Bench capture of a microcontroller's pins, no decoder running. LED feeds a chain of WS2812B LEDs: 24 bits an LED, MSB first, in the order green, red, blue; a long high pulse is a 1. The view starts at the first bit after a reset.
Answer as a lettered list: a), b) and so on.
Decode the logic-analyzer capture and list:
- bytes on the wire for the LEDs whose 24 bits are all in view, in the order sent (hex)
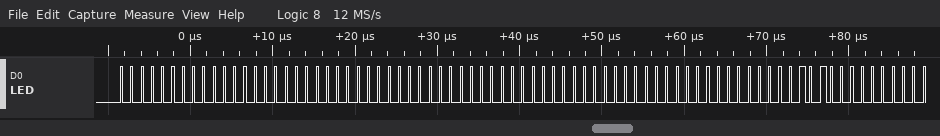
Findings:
a) 00 00 00 00 00 00 00 00 28
